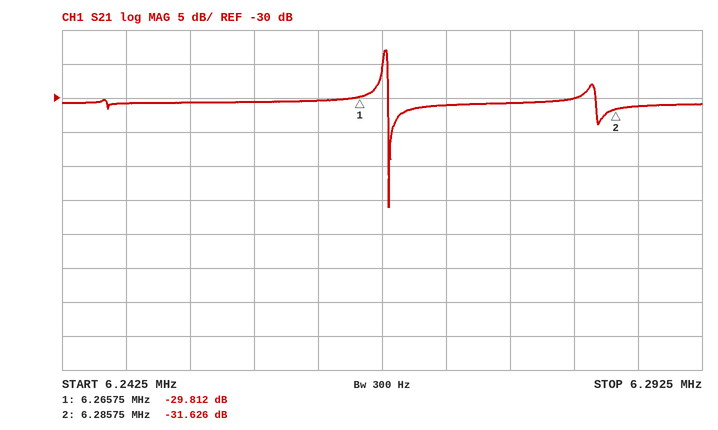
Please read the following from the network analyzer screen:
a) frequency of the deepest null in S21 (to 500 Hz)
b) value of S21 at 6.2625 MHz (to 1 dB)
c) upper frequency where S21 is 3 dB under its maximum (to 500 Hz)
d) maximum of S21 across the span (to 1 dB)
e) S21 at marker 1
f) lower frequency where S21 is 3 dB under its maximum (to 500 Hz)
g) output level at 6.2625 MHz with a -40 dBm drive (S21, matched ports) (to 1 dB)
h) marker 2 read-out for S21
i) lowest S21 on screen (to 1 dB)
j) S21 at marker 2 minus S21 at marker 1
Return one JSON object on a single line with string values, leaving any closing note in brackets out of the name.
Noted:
{"frequency of the deepest null in S21": "6.2680 MHz", "value of S21 at 6.2625 MHz": "-30 dB", "upper frequency where S21 is 3 dB under its maximum": "6.2680 MHz", "maximum of S21 across the span": "-23 dB", "S21 at marker 1": "-29.812 dB", "lower frequency where S21 is 3 dB under its maximum": "6.2675 MHz", "output level at 6.2625 MHz with a -40 dBm drive (S21, matched ports)": "-70 dBm", "marker 2 read-out for S21": "-31.626 dB", "lowest S21 on screen": "-46 dB", "S21 at marker 2 minus S21 at marker 1": "-1.814 dB"}
